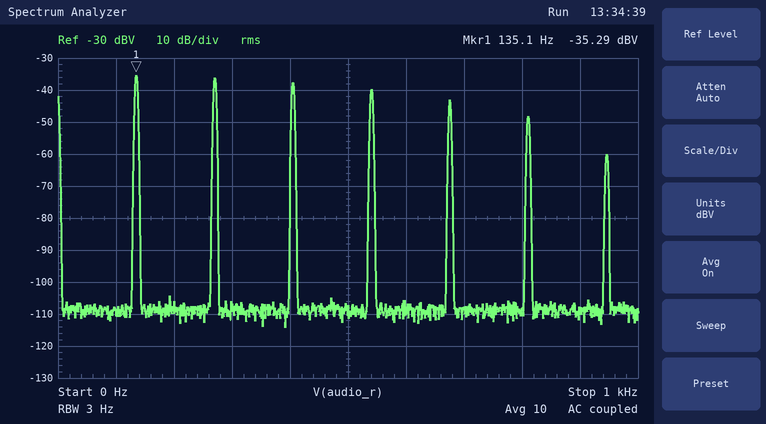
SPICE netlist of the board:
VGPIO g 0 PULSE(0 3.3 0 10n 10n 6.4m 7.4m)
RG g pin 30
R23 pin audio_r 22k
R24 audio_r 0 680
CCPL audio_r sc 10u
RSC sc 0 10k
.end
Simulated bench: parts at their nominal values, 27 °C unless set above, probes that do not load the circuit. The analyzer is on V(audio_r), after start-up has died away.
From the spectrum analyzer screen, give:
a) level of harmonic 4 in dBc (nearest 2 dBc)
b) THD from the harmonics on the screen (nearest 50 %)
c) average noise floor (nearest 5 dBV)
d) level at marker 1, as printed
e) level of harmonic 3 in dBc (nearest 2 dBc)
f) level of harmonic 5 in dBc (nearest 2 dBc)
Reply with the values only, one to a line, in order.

-4 dBc
150 %
-110 dBV
-35.29 dBV
-2 dBc
-8 dBc
